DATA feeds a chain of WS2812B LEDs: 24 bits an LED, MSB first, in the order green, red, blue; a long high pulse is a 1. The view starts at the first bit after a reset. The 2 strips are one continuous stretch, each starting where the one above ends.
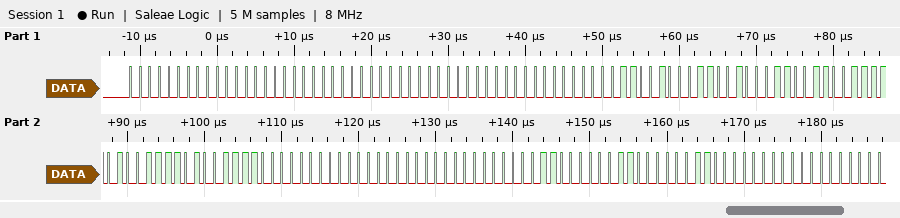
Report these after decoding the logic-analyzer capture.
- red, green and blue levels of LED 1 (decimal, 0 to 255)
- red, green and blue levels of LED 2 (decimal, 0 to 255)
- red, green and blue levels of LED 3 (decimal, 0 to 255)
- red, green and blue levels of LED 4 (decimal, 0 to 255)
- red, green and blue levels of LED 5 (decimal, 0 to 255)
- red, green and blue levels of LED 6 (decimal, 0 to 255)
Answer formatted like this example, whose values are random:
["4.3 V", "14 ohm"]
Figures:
["0, 0, 0", "0, 0, 0", "25, 25, 25", "158, 158, 158", "0, 0, 0", "12, 12, 12"]
